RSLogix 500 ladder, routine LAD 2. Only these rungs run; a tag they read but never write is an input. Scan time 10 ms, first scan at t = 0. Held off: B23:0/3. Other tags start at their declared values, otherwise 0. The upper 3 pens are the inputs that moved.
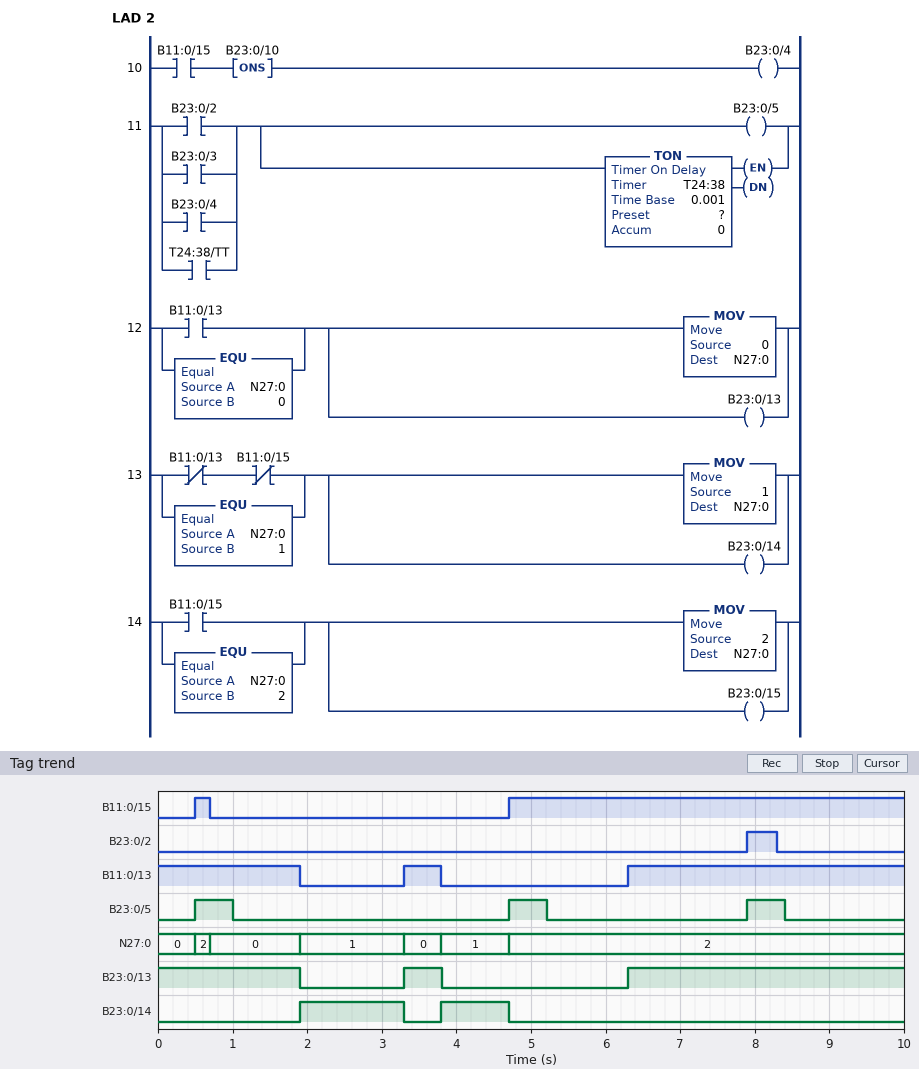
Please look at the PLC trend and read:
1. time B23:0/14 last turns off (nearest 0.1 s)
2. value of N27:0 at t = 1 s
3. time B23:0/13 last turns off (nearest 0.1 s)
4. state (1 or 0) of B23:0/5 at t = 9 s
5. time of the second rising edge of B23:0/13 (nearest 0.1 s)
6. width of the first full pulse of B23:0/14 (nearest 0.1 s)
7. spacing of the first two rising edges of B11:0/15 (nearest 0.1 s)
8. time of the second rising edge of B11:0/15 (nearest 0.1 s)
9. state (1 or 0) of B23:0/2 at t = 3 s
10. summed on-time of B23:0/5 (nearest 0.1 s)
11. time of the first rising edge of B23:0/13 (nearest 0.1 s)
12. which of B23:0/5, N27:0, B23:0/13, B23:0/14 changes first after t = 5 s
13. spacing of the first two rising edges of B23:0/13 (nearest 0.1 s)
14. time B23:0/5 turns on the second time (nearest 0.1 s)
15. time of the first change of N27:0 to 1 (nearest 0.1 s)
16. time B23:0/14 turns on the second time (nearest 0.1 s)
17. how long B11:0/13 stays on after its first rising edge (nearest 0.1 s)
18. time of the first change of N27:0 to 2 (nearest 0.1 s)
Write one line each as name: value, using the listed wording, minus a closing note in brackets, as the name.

time B23:0/14 last turns off: 4.7 s
value of N27:0 at t = 1 s: 0
time B23:0/13 last turns off: 3.8 s
state (1 or 0) of B23:0/5 at t = 9 s: 0
time of the second rising edge of B23:0/13: 6.3 s
width of the first full pulse of B23:0/14: 1.4 s
spacing of the first two rising edges of B11:0/15: 4.2 s
time of the second rising edge of B11:0/15: 4.7 s
state (1 or 0) of B23:0/2 at t = 3 s: 0
summed on-time of B23:0/5: 1.5 s
time of the first rising edge of B23:0/13: 3.3 s
which of B23:0/5, N27:0, B23:0/13, B23:0/14 changes first after t = 5 s: B23:0/5
spacing of the first two rising edges of B23:0/13: 3.0 s
time B23:0/5 turns on the second time: 4.7 s
time of the first change of N27:0 to 1: 1.9 s
time B23:0/14 turns on the second time: 3.8 s
how long B11:0/13 stays on after its first rising edge: 0.5 s
time of the first change of N27:0 to 2: 0.5 s
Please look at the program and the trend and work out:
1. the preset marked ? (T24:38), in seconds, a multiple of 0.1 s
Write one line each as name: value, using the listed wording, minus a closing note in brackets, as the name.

the preset marked ? (T24:38), in seconds, a multiple of 0.1 s: 0.5 s
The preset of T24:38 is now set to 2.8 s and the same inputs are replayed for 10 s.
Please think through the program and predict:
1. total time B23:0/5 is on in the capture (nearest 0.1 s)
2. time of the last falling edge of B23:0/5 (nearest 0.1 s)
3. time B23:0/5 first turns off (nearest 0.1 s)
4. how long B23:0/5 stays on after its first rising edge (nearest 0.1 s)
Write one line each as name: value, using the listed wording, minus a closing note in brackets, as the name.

total time B23:0/5 is on in the capture: 7.7 s
time of the last falling edge of B23:0/5: 7.5 s
time B23:0/5 first turns off: 3.3 s
how long B23:0/5 stays on after its first rising edge: 2.8 s
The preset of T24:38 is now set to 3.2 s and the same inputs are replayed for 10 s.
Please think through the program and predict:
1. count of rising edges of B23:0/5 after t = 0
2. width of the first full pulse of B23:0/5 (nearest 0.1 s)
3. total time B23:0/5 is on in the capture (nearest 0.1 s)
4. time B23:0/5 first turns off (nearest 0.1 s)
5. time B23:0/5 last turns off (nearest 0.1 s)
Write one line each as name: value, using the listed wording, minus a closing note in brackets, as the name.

count of rising edges of B23:0/5 after t = 0: 2
width of the first full pulse of B23:0/5: 3.2 s
total time B23:0/5 is on in the capture: 6.8 s
time B23:0/5 first turns off: 3.7 s
time B23:0/5 last turns off: 8.3 s
